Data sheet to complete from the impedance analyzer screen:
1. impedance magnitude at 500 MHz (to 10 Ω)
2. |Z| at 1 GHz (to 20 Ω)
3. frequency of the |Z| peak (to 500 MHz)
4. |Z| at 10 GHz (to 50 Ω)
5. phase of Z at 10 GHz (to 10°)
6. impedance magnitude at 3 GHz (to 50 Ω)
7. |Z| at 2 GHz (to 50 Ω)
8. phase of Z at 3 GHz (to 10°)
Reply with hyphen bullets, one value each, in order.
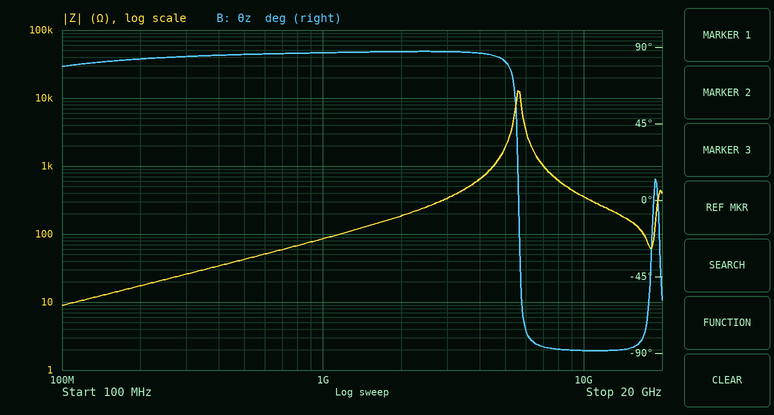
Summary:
- 40 Ω
- 80 Ω
- 5.5 GHz
- 350 Ω
- -90°
- 350 Ω
- 200 Ω
- 90°
